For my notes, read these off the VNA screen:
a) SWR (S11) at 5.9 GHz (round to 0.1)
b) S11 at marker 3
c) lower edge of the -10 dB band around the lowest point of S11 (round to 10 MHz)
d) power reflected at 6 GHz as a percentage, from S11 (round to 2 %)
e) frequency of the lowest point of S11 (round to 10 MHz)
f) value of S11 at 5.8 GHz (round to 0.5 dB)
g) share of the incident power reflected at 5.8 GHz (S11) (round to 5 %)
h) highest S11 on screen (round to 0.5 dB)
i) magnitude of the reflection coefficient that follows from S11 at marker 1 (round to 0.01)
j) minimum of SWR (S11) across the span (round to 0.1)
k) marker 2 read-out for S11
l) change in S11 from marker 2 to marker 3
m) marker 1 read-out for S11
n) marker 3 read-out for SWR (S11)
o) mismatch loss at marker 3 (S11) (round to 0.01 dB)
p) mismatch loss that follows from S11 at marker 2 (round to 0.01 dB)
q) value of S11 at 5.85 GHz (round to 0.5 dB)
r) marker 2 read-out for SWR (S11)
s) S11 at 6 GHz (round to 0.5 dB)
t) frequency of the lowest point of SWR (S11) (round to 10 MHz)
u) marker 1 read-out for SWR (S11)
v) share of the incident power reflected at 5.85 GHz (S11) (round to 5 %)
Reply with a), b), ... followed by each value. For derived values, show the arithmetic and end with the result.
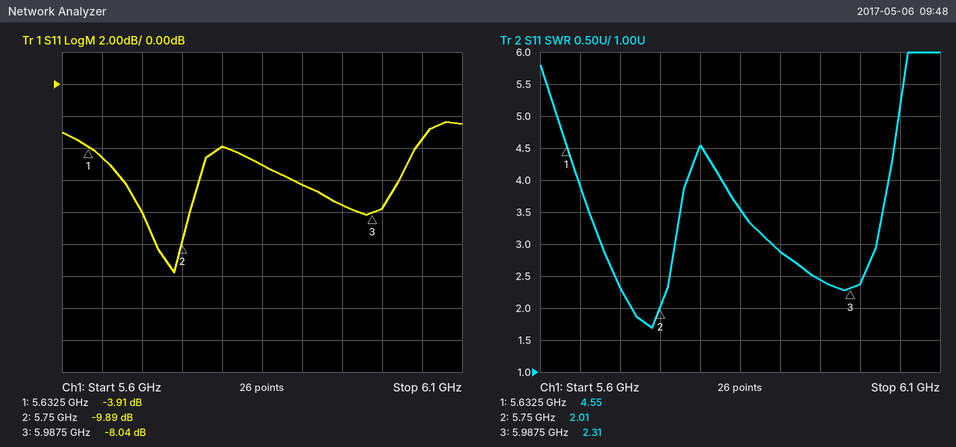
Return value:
a) 2.9
b) -8.04 dB
c) 5.72 GHz
d) 10^(-8/10) ≈ 16 %
e) 5.74 GHz
f) -4.0 dB
g) 10^(-4/10) ≈ 40 %
h) -2.5 dB
i) 10^(-3.91/20) ≈ 0.64
j) 1.7
k) -9.89 dB
l) -8.04 − (-9.89) = 1.85 dB
m) -3.91 dB
n) 2.31
o) −10 log10(1 − 10^(-8.04/10)) ≈ 0.74 dB
p) −10 log10(1 − 10^(-9.89/10)) ≈ 0.47 dB
q) -5.0 dB
r) 2.01
s) -8.0 dB
t) 5.74 GHz
u) 4.55
v) 10^(-5/10) ≈ 31.6 %, so 30 % to the nearest 5 %
